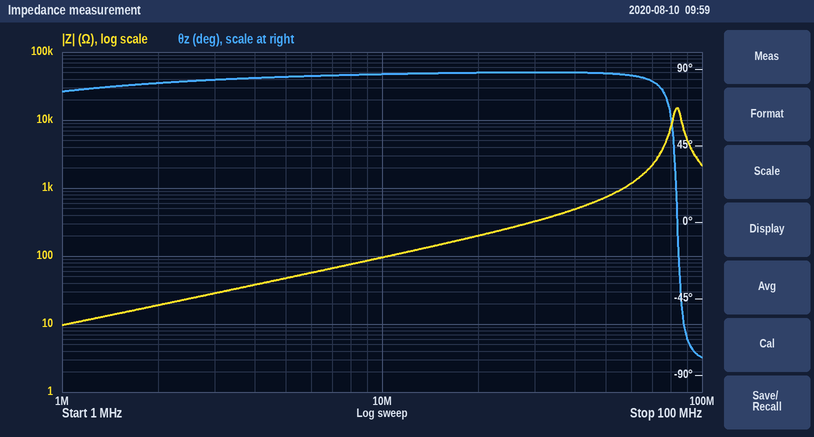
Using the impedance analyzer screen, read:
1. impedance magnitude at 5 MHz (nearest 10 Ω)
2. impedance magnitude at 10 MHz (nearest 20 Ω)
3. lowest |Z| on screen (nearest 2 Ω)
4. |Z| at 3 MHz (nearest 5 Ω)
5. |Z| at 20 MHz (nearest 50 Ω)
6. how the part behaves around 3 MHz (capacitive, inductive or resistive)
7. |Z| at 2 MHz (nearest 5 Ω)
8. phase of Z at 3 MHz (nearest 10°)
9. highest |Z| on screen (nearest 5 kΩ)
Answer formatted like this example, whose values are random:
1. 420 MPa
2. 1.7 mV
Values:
1. 50 Ω
2. 100 Ω
3. 10 Ω
4. 30 Ω
5. 200 Ω
6. inductive
7. 20 Ω
8. 80°
9. 15 kΩ
